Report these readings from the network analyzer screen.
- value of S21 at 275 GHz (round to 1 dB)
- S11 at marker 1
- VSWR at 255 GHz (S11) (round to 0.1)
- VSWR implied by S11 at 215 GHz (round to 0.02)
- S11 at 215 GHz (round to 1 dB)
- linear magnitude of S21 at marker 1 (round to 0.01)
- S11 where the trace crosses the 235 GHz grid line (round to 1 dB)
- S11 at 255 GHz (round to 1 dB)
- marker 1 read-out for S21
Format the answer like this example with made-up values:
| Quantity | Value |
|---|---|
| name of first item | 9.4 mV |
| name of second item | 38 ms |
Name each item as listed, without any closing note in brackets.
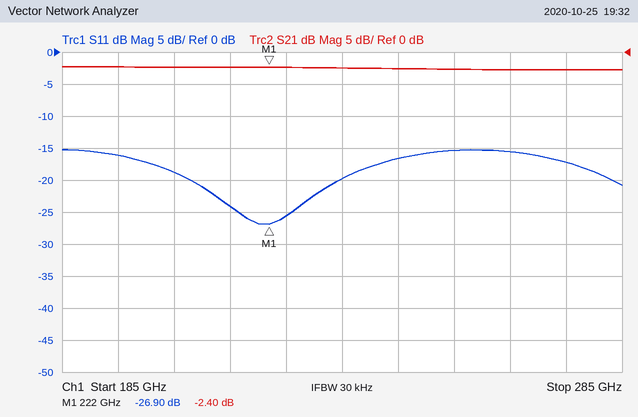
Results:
| Quantity | Value |
|---|---|
| value of S21 at 275 GHz | -3 dB |
| S11 at marker 1 | -26.90 dB |
| VSWR at 255 GHz (S11) | 1.4 |
| VSWR implied by S11 at 215 GHz | 1.14 |
| S11 at 215 GHz | -24 dB |
| linear magnitude of S21 at marker 1 | 0.76 |
| S11 where the trace crosses the 235 GHz grid line | -20 dB |
| S11 at 255 GHz | -15 dB |
| marker 1 read-out for S21 | -2.40 dB |
